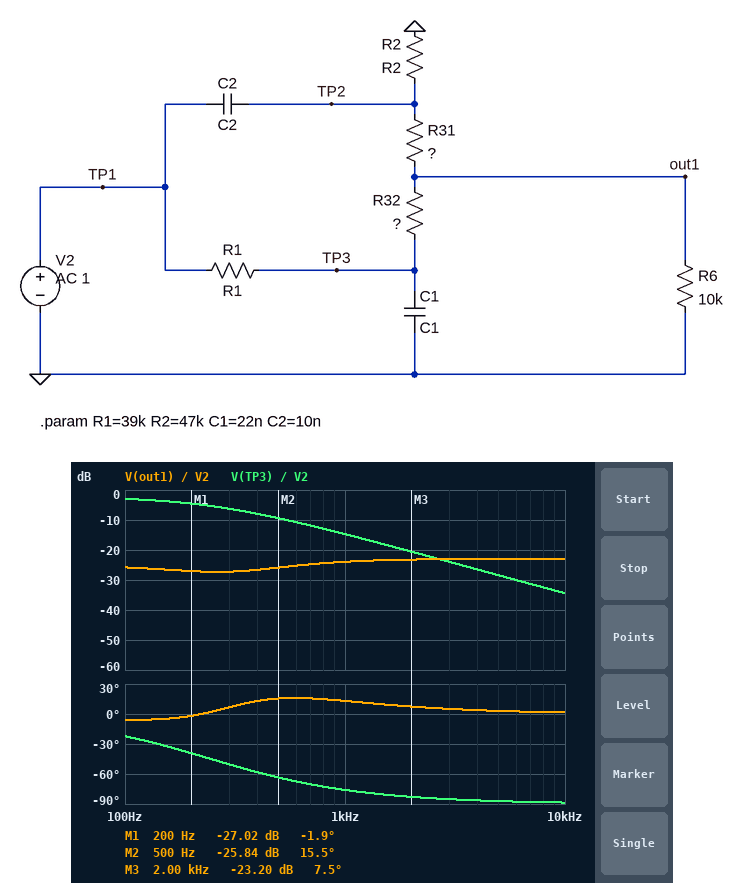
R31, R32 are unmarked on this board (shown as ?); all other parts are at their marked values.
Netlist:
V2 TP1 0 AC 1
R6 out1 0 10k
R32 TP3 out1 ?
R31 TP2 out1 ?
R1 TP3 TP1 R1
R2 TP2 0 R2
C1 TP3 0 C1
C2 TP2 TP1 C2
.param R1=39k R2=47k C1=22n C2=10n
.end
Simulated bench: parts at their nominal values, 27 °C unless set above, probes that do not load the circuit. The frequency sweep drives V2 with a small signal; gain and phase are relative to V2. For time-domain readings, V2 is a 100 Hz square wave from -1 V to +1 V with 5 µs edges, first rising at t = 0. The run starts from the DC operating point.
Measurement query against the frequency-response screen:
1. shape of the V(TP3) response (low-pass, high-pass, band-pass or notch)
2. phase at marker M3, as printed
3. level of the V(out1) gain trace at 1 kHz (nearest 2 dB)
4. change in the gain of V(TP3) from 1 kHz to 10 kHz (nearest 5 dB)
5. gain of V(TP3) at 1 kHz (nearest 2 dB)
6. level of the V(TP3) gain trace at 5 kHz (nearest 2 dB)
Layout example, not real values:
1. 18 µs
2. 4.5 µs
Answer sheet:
1. low-pass
2. 7.5 deg
3. -24 dB
4. -20 dB
5. -14 dB
6. -28 dB
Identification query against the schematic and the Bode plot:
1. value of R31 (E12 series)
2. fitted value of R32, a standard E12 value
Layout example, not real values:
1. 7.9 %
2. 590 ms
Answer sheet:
1. 120 kΩ
2. 120 kΩ
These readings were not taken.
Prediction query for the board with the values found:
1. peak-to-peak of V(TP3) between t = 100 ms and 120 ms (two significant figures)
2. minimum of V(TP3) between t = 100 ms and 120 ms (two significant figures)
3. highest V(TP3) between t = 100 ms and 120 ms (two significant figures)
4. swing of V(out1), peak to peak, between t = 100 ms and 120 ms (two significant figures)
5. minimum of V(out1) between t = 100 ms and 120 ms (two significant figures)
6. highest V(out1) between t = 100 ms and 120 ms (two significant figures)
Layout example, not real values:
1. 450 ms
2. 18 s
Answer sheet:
1. 1.5 V
2. -770 mV
3. 770 mV
4. 170 mV
5. -86 mV
6. 86 mV
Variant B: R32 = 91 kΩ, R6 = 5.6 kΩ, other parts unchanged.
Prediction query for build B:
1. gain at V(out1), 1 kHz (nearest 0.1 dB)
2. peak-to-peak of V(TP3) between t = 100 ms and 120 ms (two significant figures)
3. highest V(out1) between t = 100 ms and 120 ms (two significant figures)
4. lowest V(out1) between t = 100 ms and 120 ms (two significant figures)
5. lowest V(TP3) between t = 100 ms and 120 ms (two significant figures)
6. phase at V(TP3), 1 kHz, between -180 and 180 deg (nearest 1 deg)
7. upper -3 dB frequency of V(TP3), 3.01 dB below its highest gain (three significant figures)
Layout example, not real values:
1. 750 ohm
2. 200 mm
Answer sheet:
1. -28.5 dB
2. 1.4 V
3. 44 mV
4. -44 mV
5. -710 mV
6. -75 deg
7. 263 Hz
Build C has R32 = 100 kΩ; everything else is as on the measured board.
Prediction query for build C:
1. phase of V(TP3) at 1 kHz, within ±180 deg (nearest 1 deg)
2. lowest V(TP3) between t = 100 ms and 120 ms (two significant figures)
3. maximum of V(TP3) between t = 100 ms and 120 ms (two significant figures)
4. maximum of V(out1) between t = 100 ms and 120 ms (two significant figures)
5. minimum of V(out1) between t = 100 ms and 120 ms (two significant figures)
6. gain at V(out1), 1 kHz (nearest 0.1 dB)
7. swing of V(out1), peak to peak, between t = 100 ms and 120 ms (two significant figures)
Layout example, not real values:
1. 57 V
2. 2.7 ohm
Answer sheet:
1. -75 deg
2. -740 mV
3. 740 mV
4. 77 mV
5. -77 mV
6. -24.0 dB
7. 150 mV
